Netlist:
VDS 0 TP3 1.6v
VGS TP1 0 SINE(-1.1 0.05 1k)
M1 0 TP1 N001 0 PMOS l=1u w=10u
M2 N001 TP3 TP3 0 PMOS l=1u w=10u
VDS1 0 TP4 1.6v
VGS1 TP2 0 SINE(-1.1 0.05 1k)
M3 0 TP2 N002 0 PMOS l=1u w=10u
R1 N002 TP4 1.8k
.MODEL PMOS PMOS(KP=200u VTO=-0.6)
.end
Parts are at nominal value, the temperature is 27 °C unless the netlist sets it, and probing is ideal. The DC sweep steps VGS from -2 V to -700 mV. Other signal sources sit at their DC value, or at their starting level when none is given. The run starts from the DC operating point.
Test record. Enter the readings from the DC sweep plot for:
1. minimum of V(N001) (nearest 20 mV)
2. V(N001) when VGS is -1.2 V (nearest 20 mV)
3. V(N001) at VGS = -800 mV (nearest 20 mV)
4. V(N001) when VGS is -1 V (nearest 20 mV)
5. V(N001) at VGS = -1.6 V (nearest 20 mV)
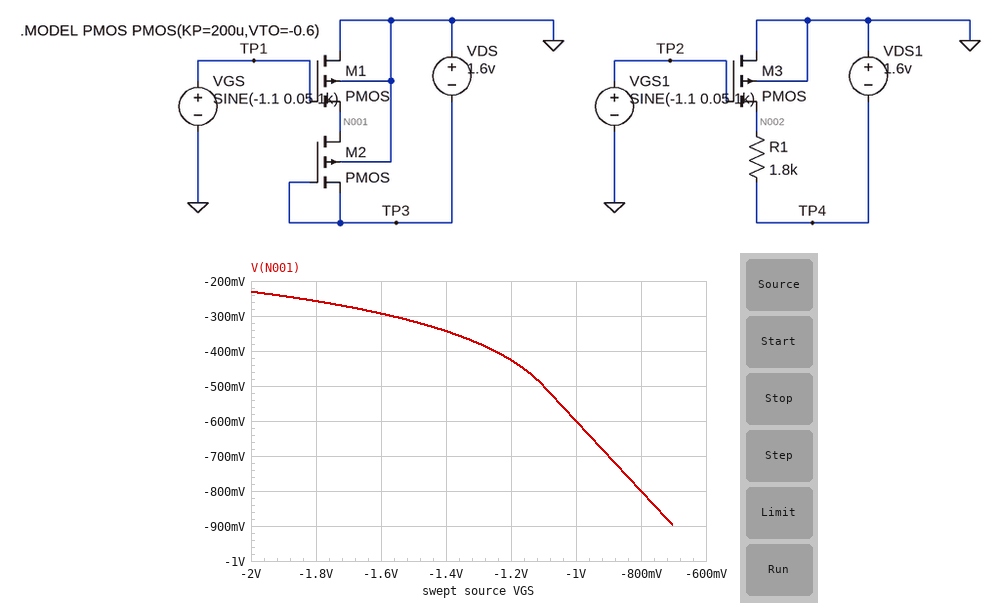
-900 mV
-420 mV
-800 mV
-600 mV
-300 mV
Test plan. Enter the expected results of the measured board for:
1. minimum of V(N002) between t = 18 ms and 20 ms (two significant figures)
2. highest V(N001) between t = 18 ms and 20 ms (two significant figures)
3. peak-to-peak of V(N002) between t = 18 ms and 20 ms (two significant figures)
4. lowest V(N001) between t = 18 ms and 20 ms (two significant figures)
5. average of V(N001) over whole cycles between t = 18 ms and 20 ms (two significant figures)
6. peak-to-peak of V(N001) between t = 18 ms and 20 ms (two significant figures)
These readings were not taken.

-1.2 V
-460 mV
180 mV
-550 mV
-500 mV
92 mV
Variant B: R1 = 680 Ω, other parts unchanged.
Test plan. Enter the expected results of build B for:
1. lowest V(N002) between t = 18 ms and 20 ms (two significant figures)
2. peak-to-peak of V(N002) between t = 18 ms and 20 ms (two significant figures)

-1.5 V
68 mV
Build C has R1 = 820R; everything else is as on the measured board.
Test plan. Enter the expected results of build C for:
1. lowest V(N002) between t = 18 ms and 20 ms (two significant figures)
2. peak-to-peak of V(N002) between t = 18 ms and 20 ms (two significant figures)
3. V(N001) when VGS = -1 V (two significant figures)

-1.4 V
82 mV
-600 mV
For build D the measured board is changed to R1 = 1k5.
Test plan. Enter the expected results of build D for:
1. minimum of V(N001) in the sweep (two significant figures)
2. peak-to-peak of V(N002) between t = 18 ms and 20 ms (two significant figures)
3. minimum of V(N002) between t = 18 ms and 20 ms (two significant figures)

-900 mV
150 mV
-1.3 V
